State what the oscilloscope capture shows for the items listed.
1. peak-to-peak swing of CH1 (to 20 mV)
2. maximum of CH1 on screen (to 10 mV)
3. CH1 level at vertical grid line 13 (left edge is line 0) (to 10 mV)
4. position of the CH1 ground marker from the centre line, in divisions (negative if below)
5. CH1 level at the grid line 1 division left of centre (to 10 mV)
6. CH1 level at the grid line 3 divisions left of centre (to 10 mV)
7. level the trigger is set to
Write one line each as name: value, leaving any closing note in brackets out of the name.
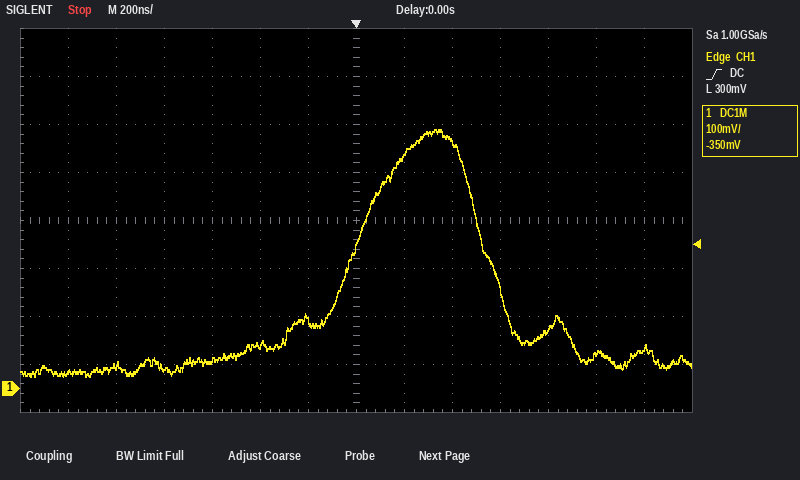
peak-to-peak swing of CH1: 520 mV
maximum of CH1 on screen: 540 mV
CH1 level at vertical grid line 13 (left edge is line 0): 80 mV
position of the CH1 ground marker from the centre line, in divisions: -3.5 div
CH1 level at the grid line 1 division left of centre: 140 mV
CH1 level at the grid line 3 divisions left of centre: 60 mV
level the trigger is set to: 300 mV
